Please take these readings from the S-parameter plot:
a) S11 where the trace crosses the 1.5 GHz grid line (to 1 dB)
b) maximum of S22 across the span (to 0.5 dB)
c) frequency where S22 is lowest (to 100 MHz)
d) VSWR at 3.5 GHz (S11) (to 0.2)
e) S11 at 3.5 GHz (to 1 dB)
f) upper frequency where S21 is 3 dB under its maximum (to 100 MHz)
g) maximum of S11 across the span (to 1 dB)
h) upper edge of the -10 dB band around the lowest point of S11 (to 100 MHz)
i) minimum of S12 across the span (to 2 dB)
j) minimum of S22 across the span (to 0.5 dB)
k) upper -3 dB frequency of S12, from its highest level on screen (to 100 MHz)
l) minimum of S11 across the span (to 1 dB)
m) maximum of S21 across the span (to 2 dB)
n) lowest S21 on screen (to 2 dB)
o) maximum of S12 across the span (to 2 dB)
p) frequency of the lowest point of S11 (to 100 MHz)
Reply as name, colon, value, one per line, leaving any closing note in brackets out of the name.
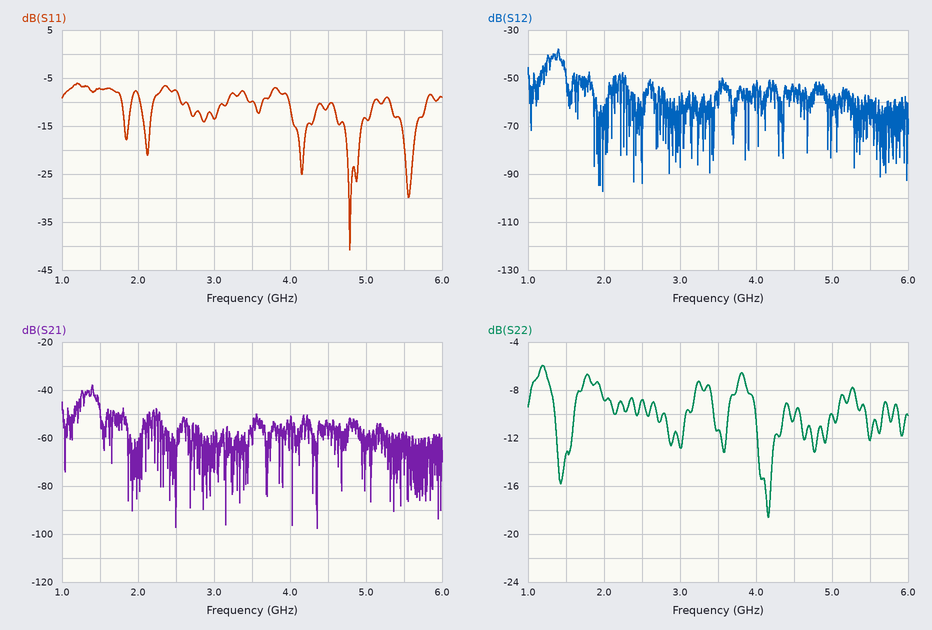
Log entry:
S11 where the trace crosses the 1.5 GHz grid line: -7 dB
maximum of S22 across the span: -6.0 dB
frequency where S22 is lowest: 4.2 GHz
VSWR at 3.5 GHz (S11): 2.0
S11 at 3.5 GHz: -10 dB
upper frequency where S21 is 3 dB under its maximum: 1.4 GHz
maximum of S11 across the span: -6 dB
upper edge of the -10 dB band around the lowest point of S11: 5.1 GHz
minimum of S12 across the span: -98 dB
minimum of S22 across the span: -18.5 dB
upper -3 dB frequency of S12, from its highest level on screen: 1.4 GHz
minimum of S11 across the span: -41 dB
maximum of S21 across the span: -38 dB
lowest S21 on screen: -98 dB
maximum of S12 across the span: -38 dB
frequency of the lowest point of S11: 4.8 GHz
